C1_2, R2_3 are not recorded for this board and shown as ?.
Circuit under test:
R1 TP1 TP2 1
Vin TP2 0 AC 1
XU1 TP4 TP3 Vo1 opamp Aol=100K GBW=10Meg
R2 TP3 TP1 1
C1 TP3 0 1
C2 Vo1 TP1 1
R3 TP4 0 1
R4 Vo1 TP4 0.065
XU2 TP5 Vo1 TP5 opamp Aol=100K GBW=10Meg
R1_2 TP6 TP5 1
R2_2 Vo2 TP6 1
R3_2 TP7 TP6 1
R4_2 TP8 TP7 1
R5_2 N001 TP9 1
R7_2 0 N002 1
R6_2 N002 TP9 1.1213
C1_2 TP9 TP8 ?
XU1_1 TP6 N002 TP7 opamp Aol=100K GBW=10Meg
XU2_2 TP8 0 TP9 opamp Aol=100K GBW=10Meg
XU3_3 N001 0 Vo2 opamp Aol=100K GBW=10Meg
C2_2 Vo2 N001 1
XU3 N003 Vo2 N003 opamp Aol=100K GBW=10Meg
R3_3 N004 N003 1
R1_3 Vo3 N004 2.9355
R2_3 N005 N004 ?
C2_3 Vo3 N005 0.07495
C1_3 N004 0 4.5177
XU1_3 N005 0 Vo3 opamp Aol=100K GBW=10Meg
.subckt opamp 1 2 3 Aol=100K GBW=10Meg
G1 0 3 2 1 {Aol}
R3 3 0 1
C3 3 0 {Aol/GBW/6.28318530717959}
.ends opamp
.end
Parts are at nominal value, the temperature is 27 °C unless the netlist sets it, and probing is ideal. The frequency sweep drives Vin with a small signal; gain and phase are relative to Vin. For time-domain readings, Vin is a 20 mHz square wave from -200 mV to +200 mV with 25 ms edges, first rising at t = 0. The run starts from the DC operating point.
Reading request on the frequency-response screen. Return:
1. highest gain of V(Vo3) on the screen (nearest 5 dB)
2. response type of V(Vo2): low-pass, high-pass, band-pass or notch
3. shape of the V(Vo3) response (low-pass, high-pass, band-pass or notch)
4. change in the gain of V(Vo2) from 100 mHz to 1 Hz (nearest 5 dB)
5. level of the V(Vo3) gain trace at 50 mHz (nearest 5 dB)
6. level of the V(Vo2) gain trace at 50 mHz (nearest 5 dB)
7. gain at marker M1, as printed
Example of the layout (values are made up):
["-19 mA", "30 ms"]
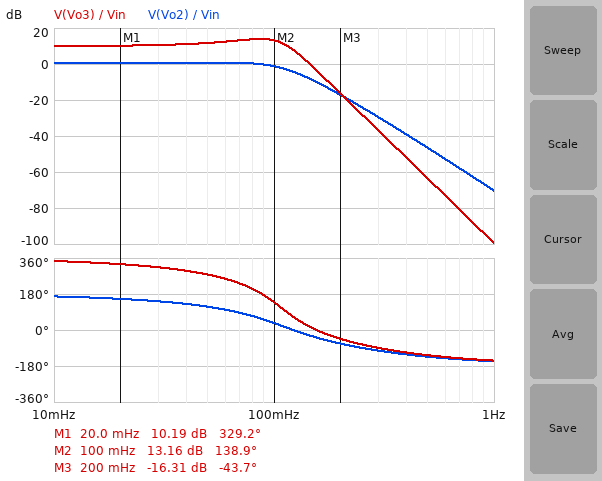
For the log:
["15 dB", "low-pass", "low-pass", "-70 dB", "10 dB", "0 dB", "10.19 dB"]
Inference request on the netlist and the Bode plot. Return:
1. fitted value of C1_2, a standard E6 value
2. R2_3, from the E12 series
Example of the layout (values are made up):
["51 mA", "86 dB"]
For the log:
["2.2 F", "2.2 Ω"]
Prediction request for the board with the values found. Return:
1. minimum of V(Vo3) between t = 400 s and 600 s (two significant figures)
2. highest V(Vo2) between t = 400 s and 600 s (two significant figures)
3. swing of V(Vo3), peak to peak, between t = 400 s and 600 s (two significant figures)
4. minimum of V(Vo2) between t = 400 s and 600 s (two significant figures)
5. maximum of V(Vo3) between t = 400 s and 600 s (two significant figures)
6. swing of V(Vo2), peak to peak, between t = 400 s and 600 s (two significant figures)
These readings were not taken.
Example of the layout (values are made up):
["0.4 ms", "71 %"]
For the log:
["-1.1 V", "260 mV", "2.2 V", "-260 mV", "1.1 V", "520 mV"]
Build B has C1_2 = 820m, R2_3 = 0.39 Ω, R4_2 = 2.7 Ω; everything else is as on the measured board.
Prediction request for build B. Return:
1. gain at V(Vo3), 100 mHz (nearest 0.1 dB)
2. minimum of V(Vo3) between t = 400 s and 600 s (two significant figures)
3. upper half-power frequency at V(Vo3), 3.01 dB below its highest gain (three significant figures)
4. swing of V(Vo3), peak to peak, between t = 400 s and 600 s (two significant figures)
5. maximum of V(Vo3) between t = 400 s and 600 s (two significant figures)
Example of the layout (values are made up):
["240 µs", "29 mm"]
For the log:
["9.4 dB", "-790 mV", "117 mHz", "1.6 V", "790 mV"]
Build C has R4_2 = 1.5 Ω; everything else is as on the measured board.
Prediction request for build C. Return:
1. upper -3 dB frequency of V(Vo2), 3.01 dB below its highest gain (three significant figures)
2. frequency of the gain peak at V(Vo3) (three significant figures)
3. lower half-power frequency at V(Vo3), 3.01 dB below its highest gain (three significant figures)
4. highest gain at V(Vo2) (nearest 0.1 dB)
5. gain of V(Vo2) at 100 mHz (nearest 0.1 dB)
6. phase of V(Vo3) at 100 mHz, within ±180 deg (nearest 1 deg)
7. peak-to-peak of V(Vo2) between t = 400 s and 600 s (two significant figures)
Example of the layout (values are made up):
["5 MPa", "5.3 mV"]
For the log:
["96.9 mHz", "79.6 mHz", "42.7 mHz", "2.1 dB", "-1.6 dB", "112 deg", "590 mV"]
